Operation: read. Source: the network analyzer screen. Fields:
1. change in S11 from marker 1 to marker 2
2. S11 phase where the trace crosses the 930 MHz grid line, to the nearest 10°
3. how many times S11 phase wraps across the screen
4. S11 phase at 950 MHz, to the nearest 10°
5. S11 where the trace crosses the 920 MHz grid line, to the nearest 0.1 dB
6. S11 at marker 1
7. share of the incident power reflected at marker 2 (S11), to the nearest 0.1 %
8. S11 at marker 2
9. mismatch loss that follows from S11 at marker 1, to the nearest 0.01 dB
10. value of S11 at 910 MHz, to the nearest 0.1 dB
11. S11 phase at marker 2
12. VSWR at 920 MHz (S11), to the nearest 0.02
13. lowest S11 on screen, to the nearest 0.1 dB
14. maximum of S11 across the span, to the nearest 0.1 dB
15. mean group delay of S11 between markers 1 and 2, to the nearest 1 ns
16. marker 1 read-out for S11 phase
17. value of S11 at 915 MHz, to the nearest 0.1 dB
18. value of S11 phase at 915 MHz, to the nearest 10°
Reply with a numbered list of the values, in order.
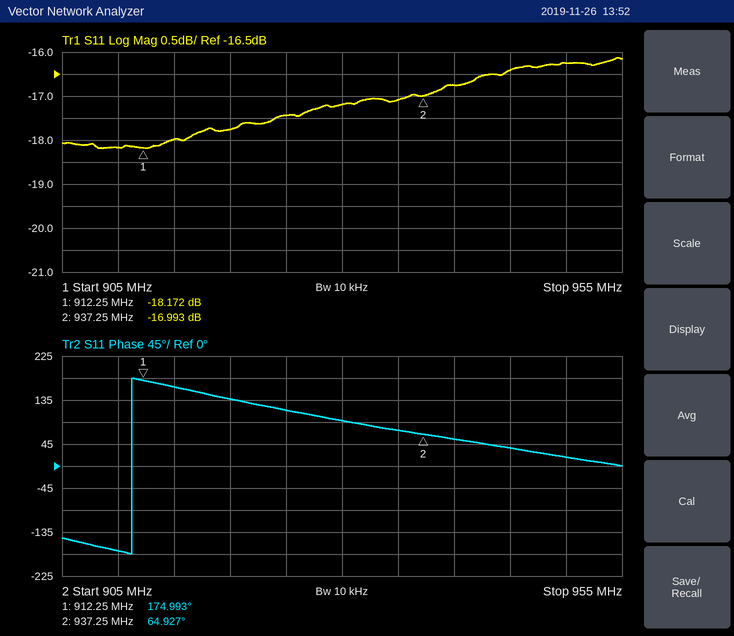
1. 1.179 dB
2. 90°
3. 1
4. 20°
5. -17.8 dB
6. -18.172 dB
7. 2.0 %
8. -16.993 dB
9. 0.07 dB
10. -18.2 dB
11. 64.927°
12. 1.30
13. -18.2 dB
14. -16.1 dB
15. 12 ns
16. 174.993°
17. -18.0 dB
18. 160°
